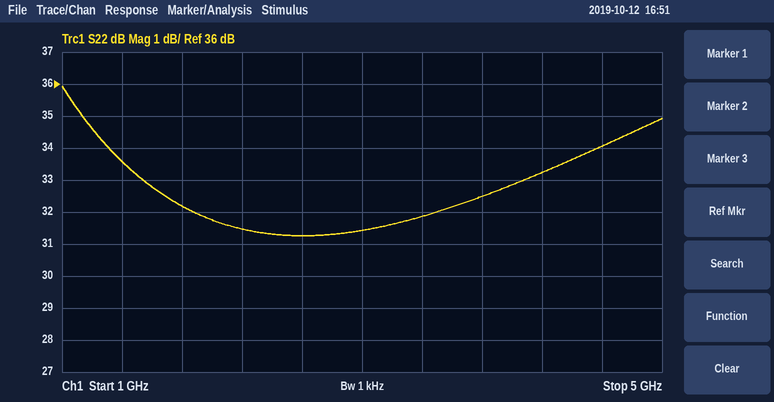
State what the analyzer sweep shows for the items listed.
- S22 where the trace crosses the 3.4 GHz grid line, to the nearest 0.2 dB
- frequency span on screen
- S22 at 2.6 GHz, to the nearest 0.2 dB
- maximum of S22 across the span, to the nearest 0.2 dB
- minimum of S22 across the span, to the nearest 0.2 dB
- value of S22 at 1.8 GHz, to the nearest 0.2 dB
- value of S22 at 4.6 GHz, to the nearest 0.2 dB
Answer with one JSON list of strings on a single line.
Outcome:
["31.8 dB", "4 GHz", "31.2 dB", "36.0 dB", "31.2 dB", "32.2 dB", "34.0 dB"]
